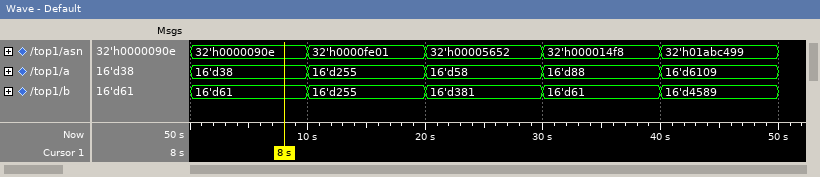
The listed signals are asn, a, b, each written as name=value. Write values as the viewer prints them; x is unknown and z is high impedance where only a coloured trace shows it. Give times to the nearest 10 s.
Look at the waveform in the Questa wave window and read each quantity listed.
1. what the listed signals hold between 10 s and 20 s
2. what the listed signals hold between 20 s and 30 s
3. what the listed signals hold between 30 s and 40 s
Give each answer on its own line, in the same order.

asn=32'h0000fe01, a=16'd255, b=16'd255
asn=32'h00005652, a=16'd58, b=16'd381
asn=32'h000014f8, a=16'd88, b=16'd61
